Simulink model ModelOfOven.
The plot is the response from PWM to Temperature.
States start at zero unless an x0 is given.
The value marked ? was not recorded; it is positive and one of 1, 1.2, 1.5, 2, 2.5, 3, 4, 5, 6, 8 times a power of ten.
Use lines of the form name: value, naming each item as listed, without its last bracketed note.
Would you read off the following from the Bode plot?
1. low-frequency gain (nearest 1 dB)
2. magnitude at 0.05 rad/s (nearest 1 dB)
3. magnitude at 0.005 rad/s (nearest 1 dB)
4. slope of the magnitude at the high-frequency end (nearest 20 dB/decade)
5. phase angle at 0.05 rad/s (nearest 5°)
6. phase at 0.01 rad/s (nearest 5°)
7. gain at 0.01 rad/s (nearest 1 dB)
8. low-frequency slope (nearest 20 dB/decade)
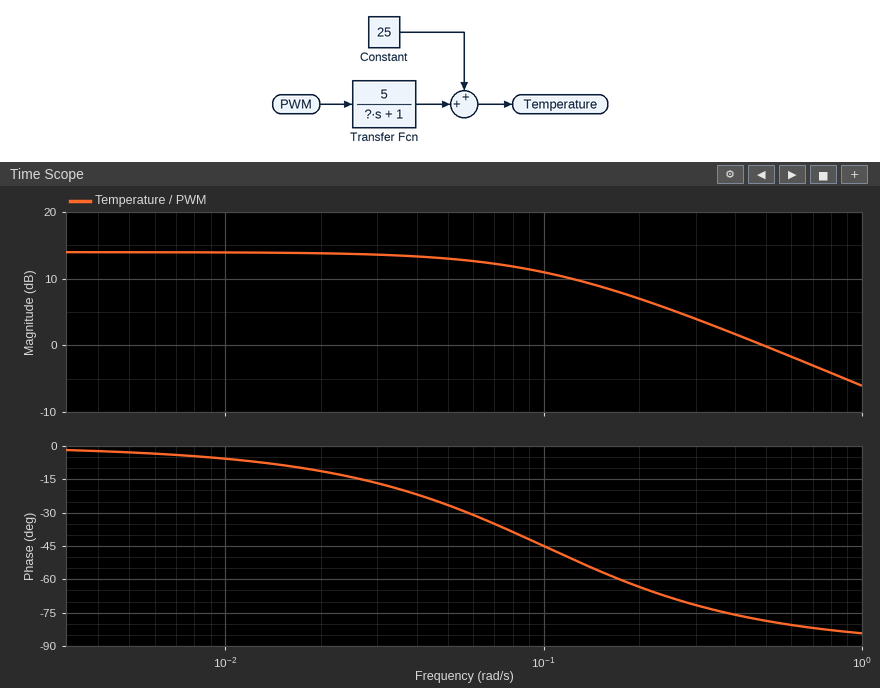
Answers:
low-frequency gain: 14 dB
magnitude at 0.05 rad/s: 13 dB
magnitude at 0.005 rad/s: 14 dB
slope of the magnitude at the high-frequency end: -20 dB/decade
phase angle at 0.05 rad/s: -25°
phase at 0.01 rad/s: -5°
gain at 0.01 rad/s: 14 dB
low-frequency slope: 0 dB/decade
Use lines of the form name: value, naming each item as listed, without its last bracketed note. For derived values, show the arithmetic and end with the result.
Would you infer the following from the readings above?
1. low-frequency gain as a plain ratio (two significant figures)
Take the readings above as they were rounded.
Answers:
low-frequency gain as a plain ratio: 10^(14 / 20) = 5.0
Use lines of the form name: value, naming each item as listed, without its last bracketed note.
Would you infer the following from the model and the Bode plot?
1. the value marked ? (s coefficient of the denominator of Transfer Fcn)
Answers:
the value marked ?: 10
